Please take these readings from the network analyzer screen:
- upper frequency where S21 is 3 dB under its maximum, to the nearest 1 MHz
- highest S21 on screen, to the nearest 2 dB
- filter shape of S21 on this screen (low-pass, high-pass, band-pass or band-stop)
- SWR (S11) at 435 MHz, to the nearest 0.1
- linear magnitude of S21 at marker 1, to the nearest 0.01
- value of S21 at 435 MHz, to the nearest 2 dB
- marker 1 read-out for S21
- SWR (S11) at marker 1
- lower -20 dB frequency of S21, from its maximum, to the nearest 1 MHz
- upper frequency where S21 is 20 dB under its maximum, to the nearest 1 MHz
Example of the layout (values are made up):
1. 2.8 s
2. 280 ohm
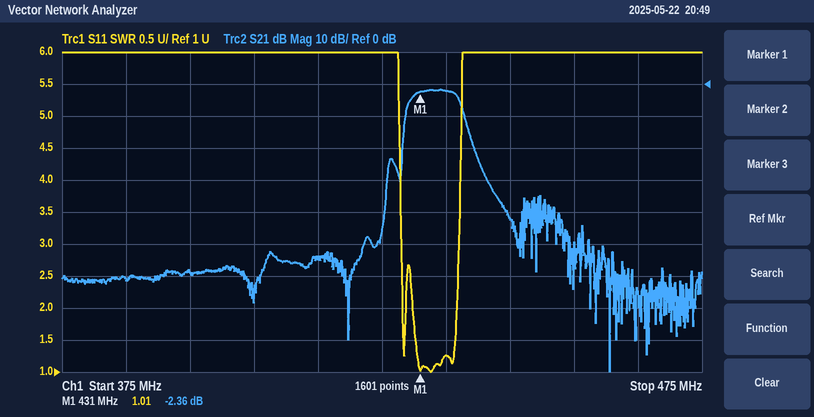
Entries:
1. 437 MHz
2. -2 dB
3. band-pass
4. 1.3
5. 0.76
6. -2 dB
7. -2.36 dB
8. 1.01
9. 428 MHz
10. 440 MHz
